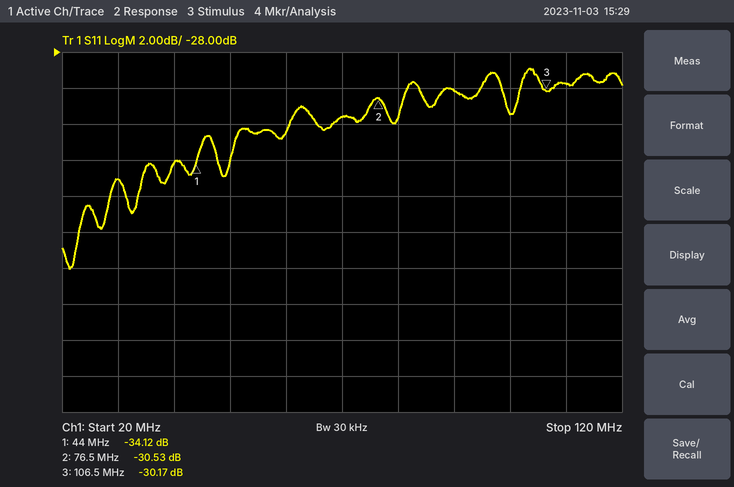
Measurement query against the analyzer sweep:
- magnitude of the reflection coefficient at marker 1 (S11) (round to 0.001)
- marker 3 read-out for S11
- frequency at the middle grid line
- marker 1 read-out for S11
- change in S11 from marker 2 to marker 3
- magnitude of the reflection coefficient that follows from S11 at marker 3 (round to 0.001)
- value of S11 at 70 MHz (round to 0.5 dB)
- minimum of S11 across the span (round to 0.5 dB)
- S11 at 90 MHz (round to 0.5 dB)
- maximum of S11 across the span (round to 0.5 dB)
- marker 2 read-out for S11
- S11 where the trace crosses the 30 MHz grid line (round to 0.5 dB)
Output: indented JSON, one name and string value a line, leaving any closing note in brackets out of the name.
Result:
{
  "magnitude of the reflection coefficient at marker 1 (S11)": "0.020",
  "marker 3 read-out for S11": "-30.17 dB",
  "frequency at the middle grid line": "70 MHz",
  "marker 1 read-out for S11": "-34.12 dB",
  "change in S11 from marker 2 to marker 3": "0.36 dB",
  "magnitude of the reflection coefficient that follows from S11 at marker 3": "0.031",
  "value of S11 at 70 MHz": "-31.5 dB",
  "minimum of S11 across the span": "-40.0 dB",
  "S11 at 90 MHz": "-30.0 dB",
  "maximum of S11 across the span": "-29.0 dB",
  "marker 2 read-out for S11": "-30.53 dB",
  "S11 where the trace crosses the 30 MHz grid line": "-35.0 dB"
}
